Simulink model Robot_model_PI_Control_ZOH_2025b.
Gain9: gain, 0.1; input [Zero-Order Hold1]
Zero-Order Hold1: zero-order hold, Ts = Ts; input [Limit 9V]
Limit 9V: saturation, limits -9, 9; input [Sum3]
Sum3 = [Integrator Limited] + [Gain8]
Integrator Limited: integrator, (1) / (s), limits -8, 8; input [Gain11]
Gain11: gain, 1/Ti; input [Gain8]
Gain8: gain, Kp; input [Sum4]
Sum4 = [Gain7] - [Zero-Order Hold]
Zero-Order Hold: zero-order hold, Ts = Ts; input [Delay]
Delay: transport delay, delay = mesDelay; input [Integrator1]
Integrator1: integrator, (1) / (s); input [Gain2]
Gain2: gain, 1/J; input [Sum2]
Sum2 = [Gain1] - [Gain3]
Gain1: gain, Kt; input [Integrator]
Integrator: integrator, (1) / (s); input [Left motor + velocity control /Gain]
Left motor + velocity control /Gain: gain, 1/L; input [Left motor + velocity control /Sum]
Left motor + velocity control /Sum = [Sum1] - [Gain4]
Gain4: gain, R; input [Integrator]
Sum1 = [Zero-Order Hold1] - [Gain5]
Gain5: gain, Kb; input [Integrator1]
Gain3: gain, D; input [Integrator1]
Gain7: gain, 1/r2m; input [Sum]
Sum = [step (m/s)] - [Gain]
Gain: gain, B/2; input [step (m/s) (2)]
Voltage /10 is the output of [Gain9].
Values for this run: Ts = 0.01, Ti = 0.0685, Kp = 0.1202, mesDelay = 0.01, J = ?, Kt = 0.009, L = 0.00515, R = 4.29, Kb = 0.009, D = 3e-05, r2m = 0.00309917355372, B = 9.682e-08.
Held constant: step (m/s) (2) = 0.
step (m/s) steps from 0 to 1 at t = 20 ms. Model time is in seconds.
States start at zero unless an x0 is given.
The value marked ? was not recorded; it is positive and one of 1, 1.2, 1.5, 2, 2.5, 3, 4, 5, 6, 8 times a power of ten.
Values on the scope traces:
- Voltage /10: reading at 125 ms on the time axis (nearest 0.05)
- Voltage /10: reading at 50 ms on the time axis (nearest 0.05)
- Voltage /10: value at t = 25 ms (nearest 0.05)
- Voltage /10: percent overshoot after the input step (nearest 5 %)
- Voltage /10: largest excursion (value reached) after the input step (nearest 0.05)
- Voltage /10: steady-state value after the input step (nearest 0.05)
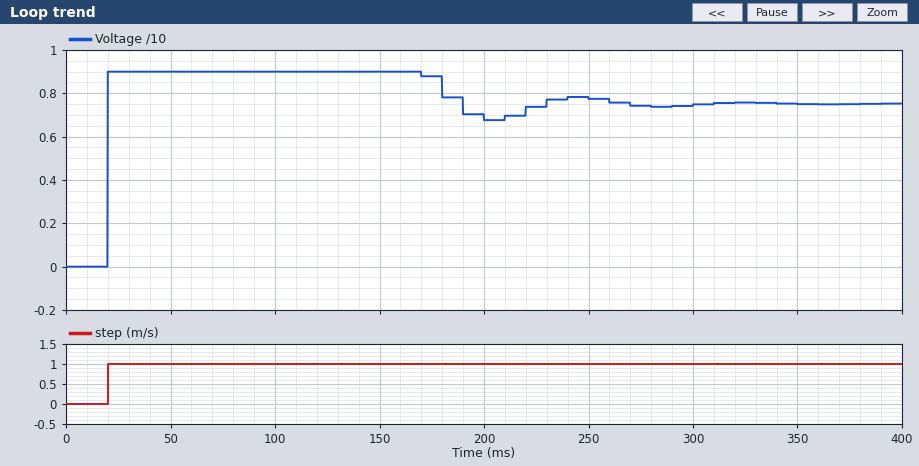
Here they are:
0.90
0.90
0.90
20 %
0.90
0.75
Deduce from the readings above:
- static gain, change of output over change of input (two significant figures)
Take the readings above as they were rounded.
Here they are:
0.75
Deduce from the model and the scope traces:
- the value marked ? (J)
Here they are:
4e-06
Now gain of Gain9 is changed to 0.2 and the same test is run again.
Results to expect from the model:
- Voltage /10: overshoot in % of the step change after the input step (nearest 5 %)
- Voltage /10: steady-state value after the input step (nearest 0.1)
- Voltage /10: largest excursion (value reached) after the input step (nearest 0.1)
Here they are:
20 %
1.5
1.8
